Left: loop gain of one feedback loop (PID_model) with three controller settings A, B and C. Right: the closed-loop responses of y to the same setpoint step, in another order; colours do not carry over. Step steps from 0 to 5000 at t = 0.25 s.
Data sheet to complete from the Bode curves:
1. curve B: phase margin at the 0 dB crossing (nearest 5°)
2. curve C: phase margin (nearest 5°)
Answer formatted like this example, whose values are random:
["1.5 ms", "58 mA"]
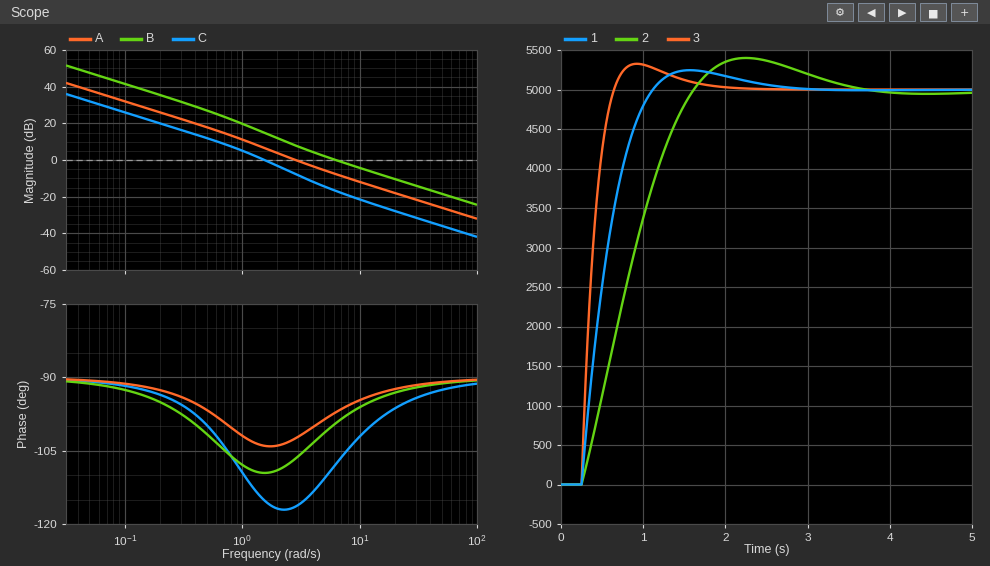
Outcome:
["80°", "65°"]
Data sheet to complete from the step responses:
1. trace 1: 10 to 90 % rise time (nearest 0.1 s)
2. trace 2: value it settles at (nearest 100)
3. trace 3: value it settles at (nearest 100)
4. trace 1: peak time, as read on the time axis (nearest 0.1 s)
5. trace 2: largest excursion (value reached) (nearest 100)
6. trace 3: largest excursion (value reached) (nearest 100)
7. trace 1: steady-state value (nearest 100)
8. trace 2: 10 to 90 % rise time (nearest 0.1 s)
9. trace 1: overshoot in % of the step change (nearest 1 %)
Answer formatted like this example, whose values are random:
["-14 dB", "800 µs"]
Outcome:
["0.6 s", "5000", "5000", "1.6 s", "5400", "5300", "5000", "1.0 s", "5 %"]
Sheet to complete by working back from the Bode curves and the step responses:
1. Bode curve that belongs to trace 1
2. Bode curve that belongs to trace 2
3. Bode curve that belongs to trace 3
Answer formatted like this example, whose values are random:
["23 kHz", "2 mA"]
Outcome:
["A", "C", "B"]
